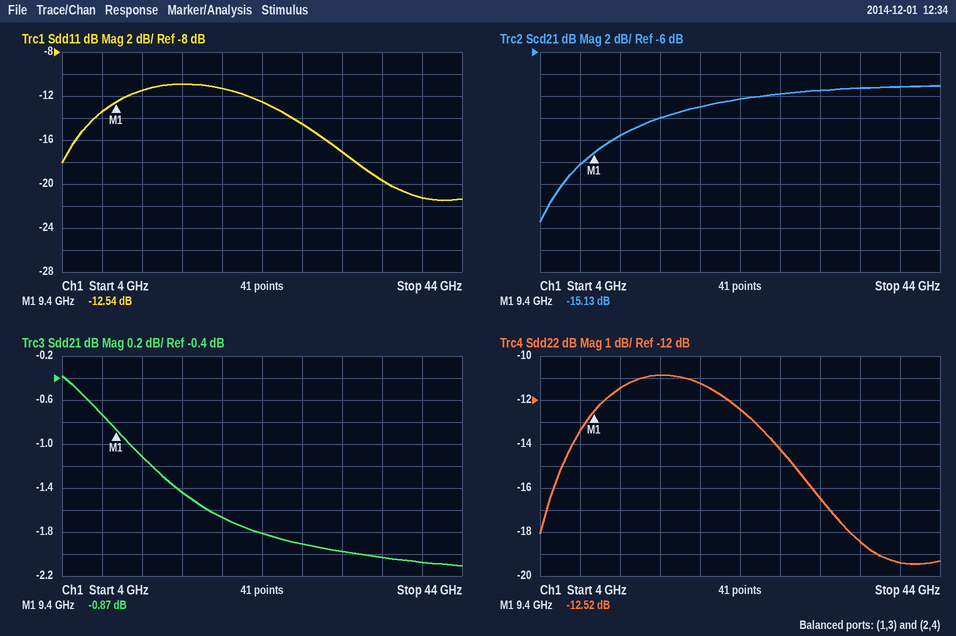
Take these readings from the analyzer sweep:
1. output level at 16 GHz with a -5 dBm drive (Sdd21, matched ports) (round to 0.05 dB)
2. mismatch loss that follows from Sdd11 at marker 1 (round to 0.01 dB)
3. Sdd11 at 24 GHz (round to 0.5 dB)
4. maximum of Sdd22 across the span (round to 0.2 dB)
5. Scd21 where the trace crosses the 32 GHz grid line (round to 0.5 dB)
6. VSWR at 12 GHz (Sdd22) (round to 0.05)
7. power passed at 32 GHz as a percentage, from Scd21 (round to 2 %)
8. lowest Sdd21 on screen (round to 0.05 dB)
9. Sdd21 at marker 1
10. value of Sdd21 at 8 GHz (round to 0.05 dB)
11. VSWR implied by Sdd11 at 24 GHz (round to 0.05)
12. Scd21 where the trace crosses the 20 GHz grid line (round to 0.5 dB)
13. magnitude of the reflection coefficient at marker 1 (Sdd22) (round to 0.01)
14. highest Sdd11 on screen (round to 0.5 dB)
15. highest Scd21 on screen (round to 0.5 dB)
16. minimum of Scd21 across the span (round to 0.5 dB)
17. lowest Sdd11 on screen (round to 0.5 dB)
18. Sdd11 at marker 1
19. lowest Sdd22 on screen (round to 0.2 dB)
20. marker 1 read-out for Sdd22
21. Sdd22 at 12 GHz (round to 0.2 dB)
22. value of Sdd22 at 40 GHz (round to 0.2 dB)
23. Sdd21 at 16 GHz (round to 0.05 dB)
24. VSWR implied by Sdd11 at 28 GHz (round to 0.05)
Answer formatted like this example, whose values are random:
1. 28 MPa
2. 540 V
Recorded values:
1. -6.45 dBm
2. 0.25 dB
3. -12.5 dB
4. -10.8 dB
5. -9.5 dB
6. 1.75
7. 12 %
8. -2.10 dB
9. -0.87 dB
10. -0.75 dB
11. 1.60
12. -11.0 dB
13. 0.24
14. -11.0 dB
15. -9.0 dB
16. -21.5 dB
17. -21.5 dB
18. -12.54 dB
19. -19.4 dB
20. -12.52 dB
21. -11.4 dB
22. -19.4 dB
23. -1.45 dB
24. 1.45
